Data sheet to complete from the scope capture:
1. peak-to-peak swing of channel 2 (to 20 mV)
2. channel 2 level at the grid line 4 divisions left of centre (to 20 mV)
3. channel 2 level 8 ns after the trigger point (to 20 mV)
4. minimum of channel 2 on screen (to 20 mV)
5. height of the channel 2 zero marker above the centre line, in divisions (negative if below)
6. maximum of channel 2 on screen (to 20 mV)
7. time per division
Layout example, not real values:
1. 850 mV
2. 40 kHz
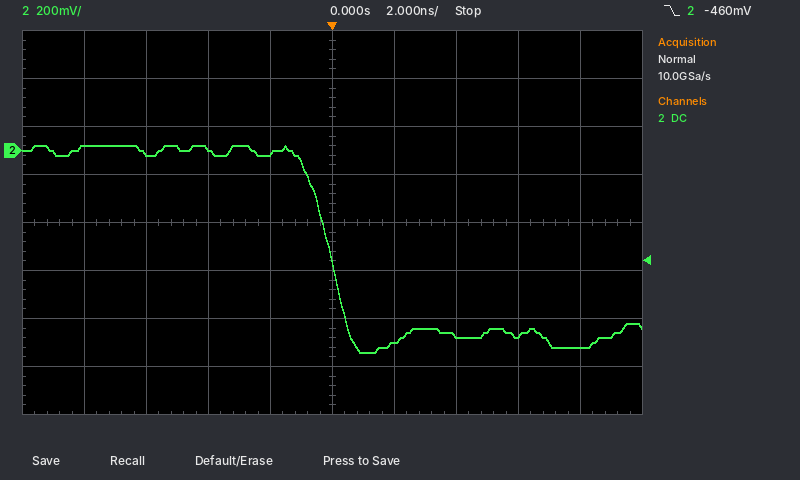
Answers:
1. 860 mV
2. 20 mV
3. -820 mV
4. -840 mV
5. +1.5 div
6. 20 mV
7. 2 ns
